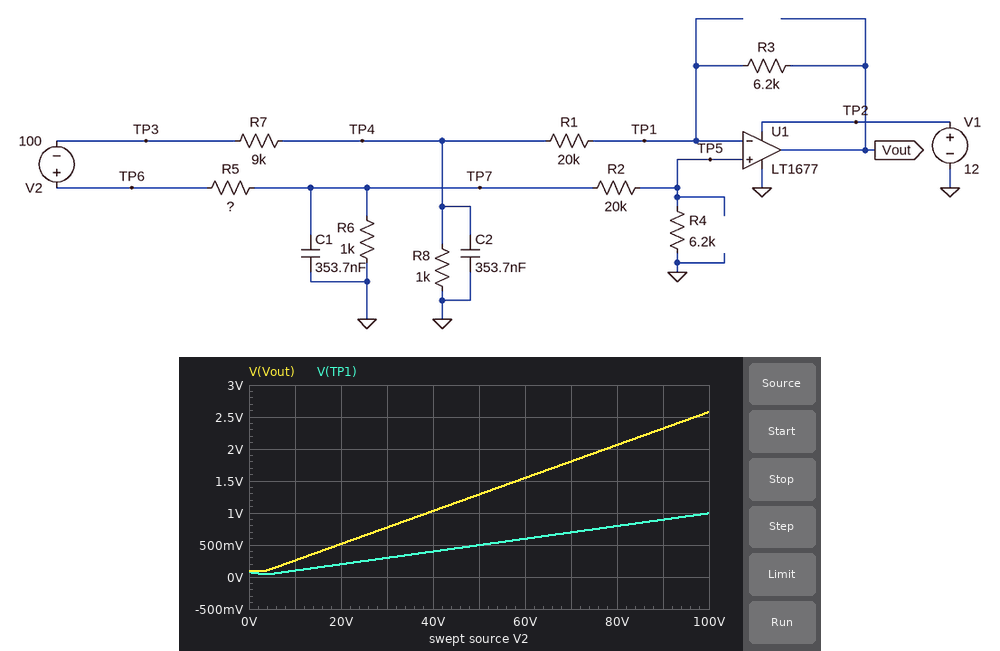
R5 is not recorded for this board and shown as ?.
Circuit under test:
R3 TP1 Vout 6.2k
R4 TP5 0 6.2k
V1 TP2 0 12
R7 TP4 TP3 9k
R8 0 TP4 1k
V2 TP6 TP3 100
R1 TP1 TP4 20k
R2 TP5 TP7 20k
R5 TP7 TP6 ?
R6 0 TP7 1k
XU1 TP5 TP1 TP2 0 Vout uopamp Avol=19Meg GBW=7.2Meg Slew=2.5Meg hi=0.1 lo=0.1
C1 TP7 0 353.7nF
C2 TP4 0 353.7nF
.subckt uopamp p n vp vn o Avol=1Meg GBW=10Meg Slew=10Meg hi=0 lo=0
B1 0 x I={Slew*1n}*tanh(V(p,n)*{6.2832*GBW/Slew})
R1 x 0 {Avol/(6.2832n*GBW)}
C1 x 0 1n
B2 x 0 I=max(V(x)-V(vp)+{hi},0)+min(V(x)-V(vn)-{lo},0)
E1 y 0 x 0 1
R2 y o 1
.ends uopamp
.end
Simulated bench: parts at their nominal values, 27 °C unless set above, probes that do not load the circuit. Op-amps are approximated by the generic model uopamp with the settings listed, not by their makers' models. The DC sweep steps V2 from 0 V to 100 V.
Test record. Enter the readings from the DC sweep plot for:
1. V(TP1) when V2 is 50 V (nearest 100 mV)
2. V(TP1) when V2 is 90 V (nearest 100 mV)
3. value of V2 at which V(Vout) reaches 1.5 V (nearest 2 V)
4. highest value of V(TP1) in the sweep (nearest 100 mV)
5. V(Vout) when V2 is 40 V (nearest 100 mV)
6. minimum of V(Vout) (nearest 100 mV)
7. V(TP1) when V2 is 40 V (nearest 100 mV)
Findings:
500 mV
900 mV
58 V
1.0 V
1.0 V
100 mV
400 mV
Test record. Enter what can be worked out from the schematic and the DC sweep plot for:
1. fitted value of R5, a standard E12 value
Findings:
12 kΩ
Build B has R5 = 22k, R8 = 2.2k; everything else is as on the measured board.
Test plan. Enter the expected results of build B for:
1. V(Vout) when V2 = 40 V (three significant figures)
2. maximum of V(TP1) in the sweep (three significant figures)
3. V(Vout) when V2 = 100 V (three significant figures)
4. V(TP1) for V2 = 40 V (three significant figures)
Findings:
1.07 V
672 mV
2.67 V
269 mV
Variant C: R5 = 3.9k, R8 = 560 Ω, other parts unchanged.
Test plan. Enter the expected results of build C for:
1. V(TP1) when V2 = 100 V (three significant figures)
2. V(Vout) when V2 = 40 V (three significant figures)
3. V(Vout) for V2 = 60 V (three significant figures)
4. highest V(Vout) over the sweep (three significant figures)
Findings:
1.58 V
1.29 V
1.94 V
3.23 V
